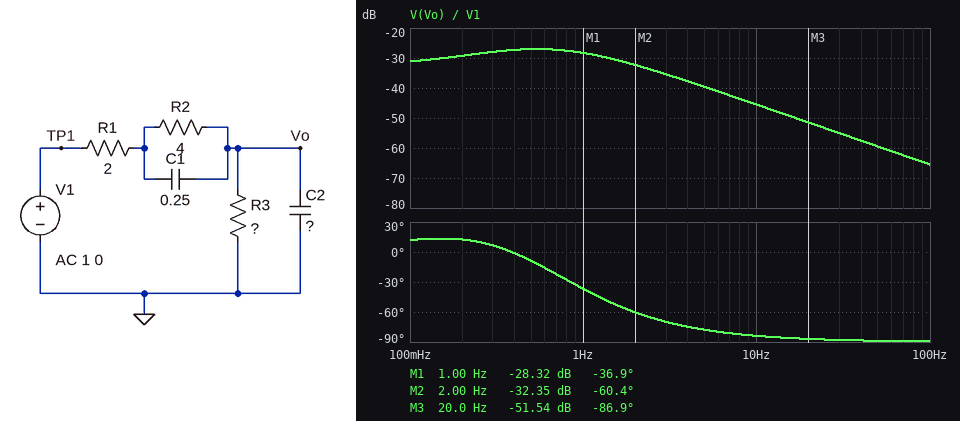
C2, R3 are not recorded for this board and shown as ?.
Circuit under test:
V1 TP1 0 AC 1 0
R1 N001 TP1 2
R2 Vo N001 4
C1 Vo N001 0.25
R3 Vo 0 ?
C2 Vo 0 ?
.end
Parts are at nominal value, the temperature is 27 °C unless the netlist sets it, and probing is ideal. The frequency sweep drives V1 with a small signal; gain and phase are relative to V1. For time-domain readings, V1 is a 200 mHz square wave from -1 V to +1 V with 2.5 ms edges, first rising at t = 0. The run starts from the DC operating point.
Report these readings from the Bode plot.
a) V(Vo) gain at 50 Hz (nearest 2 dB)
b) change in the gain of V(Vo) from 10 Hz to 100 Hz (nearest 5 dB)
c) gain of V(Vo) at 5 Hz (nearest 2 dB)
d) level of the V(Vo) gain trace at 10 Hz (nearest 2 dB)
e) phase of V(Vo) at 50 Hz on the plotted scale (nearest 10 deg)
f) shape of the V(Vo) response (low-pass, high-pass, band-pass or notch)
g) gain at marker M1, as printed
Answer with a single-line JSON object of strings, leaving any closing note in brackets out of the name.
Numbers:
{"V(Vo) gain at 50 Hz": "-60 dB", "change in the gain of V(Vo) from 10 Hz to 100 Hz": "-20 dB", "gain of V(Vo) at 5 Hz": "-40 dB", "level of the V(Vo) gain trace at 10 Hz": "-46 dB", "phase of V(Vo) at 50 Hz on the plotted scale": "-90 deg", "shape of the V(Vo) response": "low-pass", "gain at marker M1, as printed": "-28.32 dB"}
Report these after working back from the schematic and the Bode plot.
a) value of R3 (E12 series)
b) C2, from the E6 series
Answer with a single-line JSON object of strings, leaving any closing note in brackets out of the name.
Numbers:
{"value of R3": "0.15 Ω", "C2, from the E6 series": "1.5 F"}
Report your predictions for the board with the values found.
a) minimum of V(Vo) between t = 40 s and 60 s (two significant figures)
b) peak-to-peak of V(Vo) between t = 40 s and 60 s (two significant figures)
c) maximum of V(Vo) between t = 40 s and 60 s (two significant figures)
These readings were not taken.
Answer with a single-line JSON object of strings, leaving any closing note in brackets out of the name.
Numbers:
{"minimum of V(Vo) between t = 40 s and 60 s": "-55 mV", "peak-to-peak of V(Vo) between t = 40 s and 60 s": "110 mV", "maximum of V(Vo) between t = 40 s and 60 s": "55 mV"}
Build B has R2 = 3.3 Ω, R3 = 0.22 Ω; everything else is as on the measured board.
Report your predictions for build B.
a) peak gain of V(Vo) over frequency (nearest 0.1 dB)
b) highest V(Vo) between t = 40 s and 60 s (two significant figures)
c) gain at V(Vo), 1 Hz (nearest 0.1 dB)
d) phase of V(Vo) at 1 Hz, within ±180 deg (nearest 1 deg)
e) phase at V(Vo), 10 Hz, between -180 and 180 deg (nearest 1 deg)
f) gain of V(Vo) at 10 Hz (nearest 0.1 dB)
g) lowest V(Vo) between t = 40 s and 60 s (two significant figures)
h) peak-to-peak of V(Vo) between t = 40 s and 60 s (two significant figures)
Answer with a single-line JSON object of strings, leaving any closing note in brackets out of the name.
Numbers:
{"peak gain of V(Vo) over frequency": "-25.2 dB", "highest V(Vo) between t = 40 s and 60 s": "63 mV", "gain at V(Vo), 1 Hz": "-27.5 dB", "phase of V(Vo) at 1 Hz, within ±180 deg": "-46 deg", "phase at V(Vo), 10 Hz, between -180 and 180 deg": "-85 deg", "gain of V(Vo) at 10 Hz": "-45.5 dB", "lowest V(Vo) between t = 40 s and 60 s": "-63 mV", "peak-to-peak of V(Vo) between t = 40 s and 60 s": "130 mV"}
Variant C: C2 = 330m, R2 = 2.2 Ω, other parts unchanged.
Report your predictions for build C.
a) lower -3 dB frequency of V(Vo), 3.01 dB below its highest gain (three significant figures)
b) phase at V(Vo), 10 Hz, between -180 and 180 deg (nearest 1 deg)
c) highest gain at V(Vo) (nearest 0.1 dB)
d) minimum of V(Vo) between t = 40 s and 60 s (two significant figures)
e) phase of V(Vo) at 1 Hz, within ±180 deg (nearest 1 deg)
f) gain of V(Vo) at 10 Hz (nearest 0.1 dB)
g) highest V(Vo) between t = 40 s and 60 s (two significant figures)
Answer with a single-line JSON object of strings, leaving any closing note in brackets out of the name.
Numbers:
{"lower -3 dB frequency of V(Vo), 3.01 dB below its highest gain": "276 mHz", "phase at V(Vo), 10 Hz, between -180 and 180 deg": "-69 deg", "highest gain at V(Vo)": "-24.3 dB", "minimum of V(Vo) between t = 40 s and 60 s": "-78 mV", "phase of V(Vo) at 1 Hz, within ±180 deg": "-2 deg", "gain of V(Vo) at 10 Hz": "-32.9 dB", "highest V(Vo) between t = 40 s and 60 s": "78 mV"}
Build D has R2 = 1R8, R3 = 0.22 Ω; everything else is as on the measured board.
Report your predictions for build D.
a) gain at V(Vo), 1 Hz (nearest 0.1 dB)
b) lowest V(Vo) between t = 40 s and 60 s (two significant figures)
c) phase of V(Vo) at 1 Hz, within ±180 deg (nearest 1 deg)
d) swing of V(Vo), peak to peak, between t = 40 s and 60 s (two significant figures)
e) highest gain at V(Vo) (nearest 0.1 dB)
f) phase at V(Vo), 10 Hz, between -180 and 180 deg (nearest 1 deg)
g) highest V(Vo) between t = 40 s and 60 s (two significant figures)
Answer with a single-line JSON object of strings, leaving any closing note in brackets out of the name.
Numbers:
{"gain at V(Vo), 1 Hz": "-27.8 dB", "lowest V(Vo) between t = 40 s and 60 s": "-59 mV", "phase of V(Vo) at 1 Hz, within ±180 deg": "-48 deg", "swing of V(Vo), peak to peak, between t = 40 s and 60 s": "120 mV", "highest gain at V(Vo)": "-25.1 dB", "phase at V(Vo), 10 Hz, between -180 and 180 deg": "-85 deg", "highest V(Vo) between t = 40 s and 60 s": "59 mV"}
